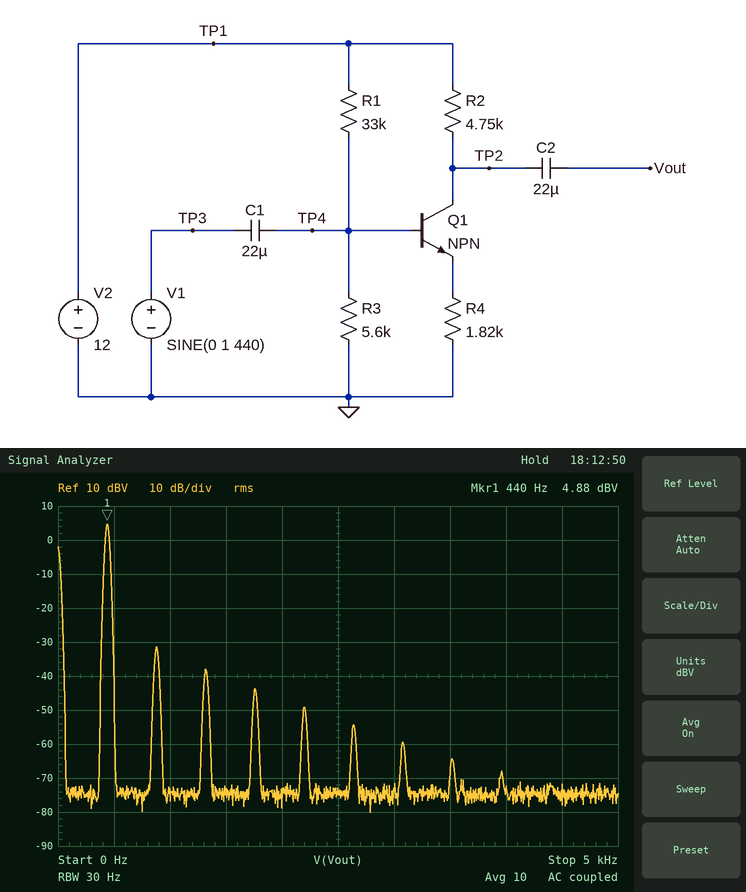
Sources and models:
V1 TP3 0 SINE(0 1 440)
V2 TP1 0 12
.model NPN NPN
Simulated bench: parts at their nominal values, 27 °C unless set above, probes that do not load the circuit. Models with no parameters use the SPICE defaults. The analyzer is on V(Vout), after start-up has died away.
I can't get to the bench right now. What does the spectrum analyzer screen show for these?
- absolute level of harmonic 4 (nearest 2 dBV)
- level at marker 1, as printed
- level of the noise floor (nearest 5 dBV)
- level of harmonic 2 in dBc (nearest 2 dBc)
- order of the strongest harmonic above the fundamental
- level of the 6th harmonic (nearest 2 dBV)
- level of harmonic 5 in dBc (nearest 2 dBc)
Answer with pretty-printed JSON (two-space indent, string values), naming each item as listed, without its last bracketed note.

{
  "absolute level of harmonic 4": "-44 dBV",
  "level at marker 1, as printed": "4.88 dBV",
  "level of the noise floor": "-75 dBV",
  "level of harmonic 2 in dBc": "-36 dBc",
  "order of the strongest harmonic above the fundamental": "2",
  "level of the 6th harmonic": "-54 dBV",
  "level of harmonic 5 in dBc": "-54 dBc"
}
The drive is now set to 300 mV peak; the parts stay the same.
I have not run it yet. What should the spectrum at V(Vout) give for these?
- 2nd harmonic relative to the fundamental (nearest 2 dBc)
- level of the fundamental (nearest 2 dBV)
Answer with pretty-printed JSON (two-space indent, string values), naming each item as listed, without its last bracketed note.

{
  "2nd harmonic relative to the fundamental": "-54 dBc",
  "level of the fundamental": "-6 dBV"
}
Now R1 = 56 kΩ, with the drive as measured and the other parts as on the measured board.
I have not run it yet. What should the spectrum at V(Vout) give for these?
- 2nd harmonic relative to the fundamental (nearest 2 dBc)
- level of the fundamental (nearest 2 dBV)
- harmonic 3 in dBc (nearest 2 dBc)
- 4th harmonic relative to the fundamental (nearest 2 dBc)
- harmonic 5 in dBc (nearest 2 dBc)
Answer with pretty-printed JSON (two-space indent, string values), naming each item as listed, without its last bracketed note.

{
  "2nd harmonic relative to the fundamental": "-12 dBc",
  "level of the fundamental": "2 dBV",
  "harmonic 3 in dBc": "-22 dBc",
  "4th harmonic relative to the fundamental": "-42 dBc",
  "harmonic 5 in dBc": "-32 dBc"
}
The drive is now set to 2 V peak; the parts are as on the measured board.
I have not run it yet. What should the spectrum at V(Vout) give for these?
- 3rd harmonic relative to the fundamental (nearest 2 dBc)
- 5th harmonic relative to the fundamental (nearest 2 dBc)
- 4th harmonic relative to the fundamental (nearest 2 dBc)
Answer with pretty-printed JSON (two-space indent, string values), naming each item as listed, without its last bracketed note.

{
  "3rd harmonic relative to the fundamental": "-22 dBc",
  "5th harmonic relative to the fundamental": "-36 dBc",
  "4th harmonic relative to the fundamental": "-36 dBc"
}
